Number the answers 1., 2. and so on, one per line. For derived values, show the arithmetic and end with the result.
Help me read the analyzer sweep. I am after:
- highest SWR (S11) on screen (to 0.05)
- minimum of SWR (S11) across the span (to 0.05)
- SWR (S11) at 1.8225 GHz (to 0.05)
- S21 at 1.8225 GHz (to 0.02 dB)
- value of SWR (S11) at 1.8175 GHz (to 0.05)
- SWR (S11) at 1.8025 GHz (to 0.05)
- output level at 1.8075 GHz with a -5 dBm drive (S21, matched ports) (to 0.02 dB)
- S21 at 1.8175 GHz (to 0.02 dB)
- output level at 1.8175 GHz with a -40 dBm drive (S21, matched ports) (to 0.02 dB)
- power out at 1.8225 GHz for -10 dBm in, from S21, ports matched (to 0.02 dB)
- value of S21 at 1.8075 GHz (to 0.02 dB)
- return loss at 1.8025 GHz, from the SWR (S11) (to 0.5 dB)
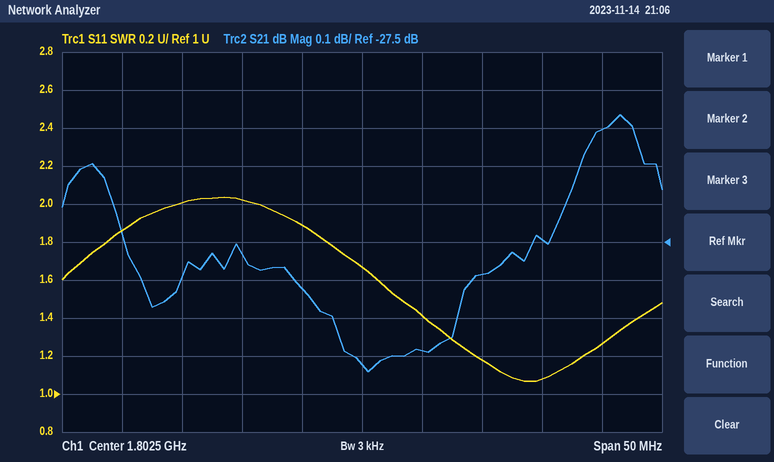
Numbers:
1. 2.05
2. 1.05
3. 1.25
4. -27.20 dB
5. 1.10
6. 1.65
7. -5 dBm + (-27.78 dB) = -32.78 dBm
8. -27.50 dB
9. -40 dBm + (-27.50 dB) = -67.50 dBm
10. -10 dBm + (-27.20 dB) = -37.20 dBm
11. -27.78 dB
12. −20 log10((1.65 − 1)/(1.65 + 1)) ≈ 12.2 dB, so 12.0 dB to the nearest 0.5 dB
